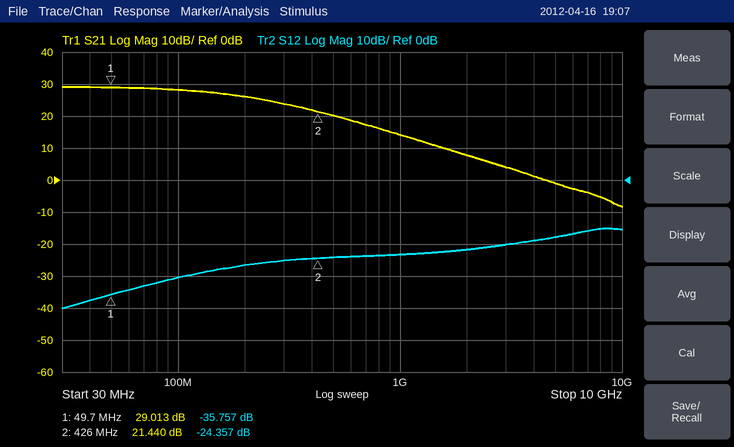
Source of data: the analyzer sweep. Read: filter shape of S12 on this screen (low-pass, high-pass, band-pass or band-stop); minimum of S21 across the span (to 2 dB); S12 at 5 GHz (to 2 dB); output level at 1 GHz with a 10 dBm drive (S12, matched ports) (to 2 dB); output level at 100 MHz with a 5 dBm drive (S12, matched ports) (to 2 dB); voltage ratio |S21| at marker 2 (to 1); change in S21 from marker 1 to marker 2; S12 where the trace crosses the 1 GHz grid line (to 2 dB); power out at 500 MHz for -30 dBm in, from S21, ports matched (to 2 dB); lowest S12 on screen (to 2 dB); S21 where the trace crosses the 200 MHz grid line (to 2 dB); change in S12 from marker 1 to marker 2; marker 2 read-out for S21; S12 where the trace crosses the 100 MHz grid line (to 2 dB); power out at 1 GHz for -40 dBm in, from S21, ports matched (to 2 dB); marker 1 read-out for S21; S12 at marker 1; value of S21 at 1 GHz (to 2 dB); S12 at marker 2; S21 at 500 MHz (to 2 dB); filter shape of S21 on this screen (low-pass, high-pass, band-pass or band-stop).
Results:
high-pass
-8 dB
-18 dB
-14 dBm
-26 dBm
12
-7.573 dB
-24 dB
-10 dBm
-40 dB
26 dB
11.400 dB
21.440 dB
-30 dB
-26 dBm
29.013 dB
-35.757 dB
14 dB
-24.357 dB
20 dB
low-pass
